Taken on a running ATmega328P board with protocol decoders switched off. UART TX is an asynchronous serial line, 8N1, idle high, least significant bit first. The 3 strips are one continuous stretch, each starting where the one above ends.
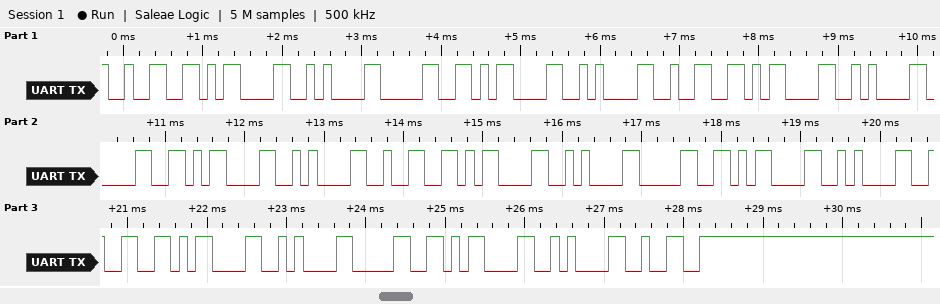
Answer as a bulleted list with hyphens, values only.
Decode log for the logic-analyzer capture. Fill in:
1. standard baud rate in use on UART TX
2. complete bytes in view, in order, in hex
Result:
- 9600 baud
- 32 0D 0A 30 0D 0A 32 0D 0A 30 0D 0A 32 0D 0A 30 0D 0A 32 0D 0A 30 0D 0A 32
